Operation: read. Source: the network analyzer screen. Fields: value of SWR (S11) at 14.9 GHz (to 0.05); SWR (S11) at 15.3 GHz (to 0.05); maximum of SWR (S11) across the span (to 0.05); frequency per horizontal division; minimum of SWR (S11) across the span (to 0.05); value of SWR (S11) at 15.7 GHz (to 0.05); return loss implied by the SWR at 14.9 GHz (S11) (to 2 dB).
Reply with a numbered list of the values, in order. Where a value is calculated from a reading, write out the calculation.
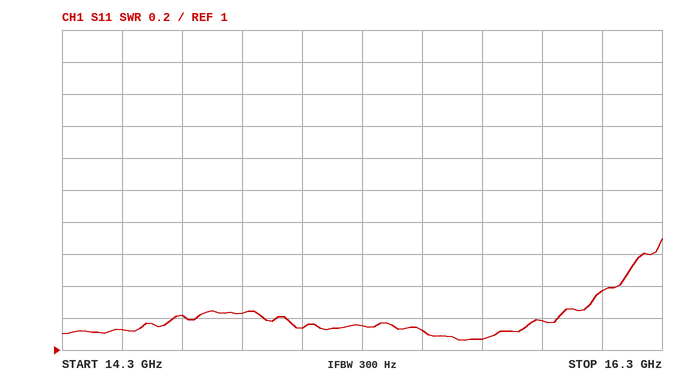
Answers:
1. 1.25
2. 1.15
3. 1.70
4. 200 MHz
5. 1.05
6. 1.05
7. −20 log10((1.25 − 1)/(1.25 + 1)) ≈ 19.1 dB, so 20 dB to the nearest 2 dB
